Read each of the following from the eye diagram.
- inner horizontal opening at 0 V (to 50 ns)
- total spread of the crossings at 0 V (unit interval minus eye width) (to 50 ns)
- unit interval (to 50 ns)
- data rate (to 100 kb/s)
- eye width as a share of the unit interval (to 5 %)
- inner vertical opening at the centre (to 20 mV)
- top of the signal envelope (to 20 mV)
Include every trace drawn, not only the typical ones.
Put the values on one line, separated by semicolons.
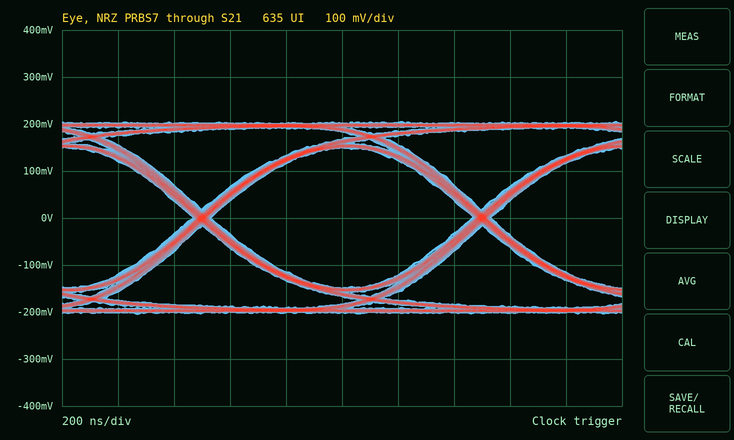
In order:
950 ns; 50 ns; 1.00 µs; 1.0 Mb/s; 95 %; 300 mV; 200 mV
